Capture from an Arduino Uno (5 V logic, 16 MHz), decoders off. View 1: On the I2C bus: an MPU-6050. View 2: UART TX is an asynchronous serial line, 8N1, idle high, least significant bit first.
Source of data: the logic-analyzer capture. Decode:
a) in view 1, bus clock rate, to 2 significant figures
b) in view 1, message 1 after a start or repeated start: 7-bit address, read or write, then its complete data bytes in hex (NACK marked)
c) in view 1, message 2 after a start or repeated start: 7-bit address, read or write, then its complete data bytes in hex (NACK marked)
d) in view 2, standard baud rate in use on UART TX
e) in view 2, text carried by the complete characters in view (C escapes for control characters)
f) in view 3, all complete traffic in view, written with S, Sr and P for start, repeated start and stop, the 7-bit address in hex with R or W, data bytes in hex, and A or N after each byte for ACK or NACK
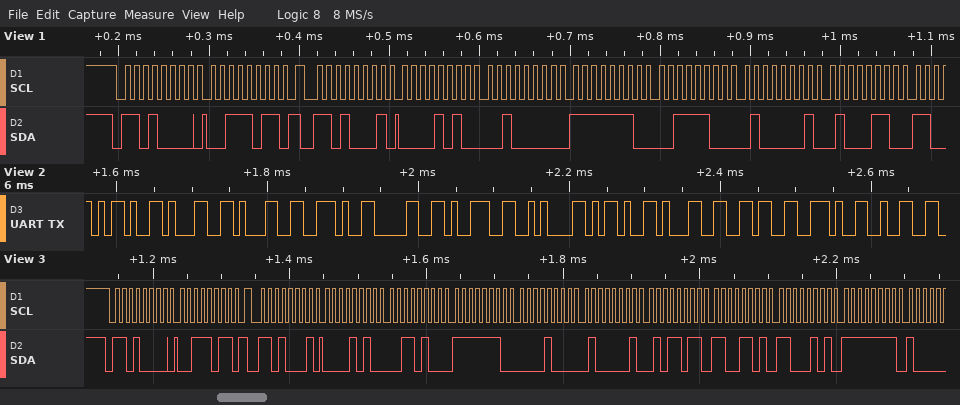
100 kHz
0x68 write: 3B
0x68 read: 0A 20 FE 3C 41 46
115200 baud
"-11.09\n-16.2"
S 68W A 3B A Sr 68R A 0A A 34 A FE A 08 A 41 A 5B A CD A C5 A FF A
